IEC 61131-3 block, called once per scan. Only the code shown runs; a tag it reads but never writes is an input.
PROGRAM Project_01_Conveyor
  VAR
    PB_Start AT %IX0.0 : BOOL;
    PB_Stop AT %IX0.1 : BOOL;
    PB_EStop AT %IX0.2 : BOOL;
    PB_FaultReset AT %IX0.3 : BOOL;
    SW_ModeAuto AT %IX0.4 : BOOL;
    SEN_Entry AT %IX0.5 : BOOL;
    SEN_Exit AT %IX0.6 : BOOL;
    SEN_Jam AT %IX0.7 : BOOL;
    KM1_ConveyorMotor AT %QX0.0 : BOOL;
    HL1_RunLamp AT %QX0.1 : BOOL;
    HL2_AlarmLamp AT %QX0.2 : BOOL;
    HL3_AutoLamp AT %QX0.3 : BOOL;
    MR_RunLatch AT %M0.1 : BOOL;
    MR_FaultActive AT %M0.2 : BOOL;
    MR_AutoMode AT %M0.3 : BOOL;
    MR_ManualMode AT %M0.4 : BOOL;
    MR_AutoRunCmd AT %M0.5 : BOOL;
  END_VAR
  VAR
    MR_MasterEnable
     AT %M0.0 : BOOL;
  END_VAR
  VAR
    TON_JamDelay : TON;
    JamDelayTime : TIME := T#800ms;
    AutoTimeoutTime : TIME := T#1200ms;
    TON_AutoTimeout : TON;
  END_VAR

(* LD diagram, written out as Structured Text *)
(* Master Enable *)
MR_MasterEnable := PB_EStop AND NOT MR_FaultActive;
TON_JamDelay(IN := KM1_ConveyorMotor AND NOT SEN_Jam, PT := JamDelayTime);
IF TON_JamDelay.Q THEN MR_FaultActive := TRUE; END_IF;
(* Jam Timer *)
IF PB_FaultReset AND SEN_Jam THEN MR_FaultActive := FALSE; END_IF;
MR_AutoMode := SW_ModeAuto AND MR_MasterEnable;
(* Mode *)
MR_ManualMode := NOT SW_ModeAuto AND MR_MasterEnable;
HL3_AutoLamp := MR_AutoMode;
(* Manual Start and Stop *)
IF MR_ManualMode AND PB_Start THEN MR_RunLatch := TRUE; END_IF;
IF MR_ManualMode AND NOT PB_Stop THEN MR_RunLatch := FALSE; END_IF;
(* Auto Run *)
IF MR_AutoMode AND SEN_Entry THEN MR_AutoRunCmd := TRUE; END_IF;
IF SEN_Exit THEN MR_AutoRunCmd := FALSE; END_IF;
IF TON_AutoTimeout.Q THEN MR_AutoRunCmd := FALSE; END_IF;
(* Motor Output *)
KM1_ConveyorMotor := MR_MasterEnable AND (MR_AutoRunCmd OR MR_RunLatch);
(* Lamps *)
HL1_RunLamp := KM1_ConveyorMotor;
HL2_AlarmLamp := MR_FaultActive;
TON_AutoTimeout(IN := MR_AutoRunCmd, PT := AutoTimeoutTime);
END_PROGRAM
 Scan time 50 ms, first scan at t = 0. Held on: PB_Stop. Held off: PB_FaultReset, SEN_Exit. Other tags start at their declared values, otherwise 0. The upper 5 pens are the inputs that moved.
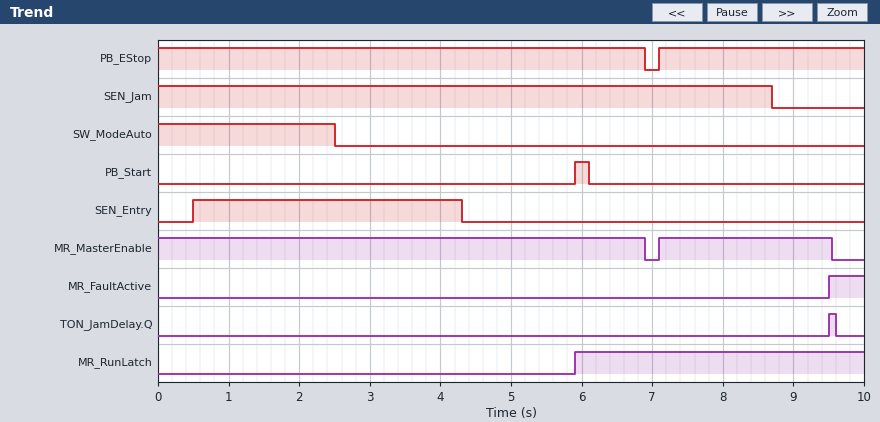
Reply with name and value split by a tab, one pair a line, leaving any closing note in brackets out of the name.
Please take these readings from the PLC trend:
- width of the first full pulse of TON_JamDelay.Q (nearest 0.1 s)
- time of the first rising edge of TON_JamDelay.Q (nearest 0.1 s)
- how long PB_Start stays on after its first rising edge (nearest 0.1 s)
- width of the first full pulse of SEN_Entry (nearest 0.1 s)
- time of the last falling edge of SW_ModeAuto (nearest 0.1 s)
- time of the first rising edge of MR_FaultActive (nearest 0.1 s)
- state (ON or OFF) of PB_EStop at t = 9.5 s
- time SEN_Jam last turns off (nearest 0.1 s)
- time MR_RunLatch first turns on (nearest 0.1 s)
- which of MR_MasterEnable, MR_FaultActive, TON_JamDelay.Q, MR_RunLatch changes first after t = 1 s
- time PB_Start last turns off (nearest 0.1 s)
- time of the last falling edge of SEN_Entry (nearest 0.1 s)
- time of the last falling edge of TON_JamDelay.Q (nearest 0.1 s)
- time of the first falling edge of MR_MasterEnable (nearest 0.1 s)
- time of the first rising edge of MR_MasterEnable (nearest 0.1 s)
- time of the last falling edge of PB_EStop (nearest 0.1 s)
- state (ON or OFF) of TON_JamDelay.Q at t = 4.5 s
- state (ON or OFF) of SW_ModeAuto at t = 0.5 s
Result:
width of the first full pulse of TON_JamDelay.Q	0.1 s
time of the first rising edge of TON_JamDelay.Q	9.5 s
how long PB_Start stays on after its first rising edge	0.2 s
width of the first full pulse of SEN_Entry	3.8 s
time of the last falling edge of SW_ModeAuto	2.5 s
time of the first rising edge of MR_FaultActive	9.5 s
state (ON or OFF) of PB_EStop at t = 9.5 s	ON
time SEN_Jam last turns off	8.7 s
time MR_RunLatch first turns on	5.9 s
which of MR_MasterEnable, MR_FaultActive, TON_JamDelay.Q, MR_RunLatch changes first after t = 1 s	MR_RunLatch
time PB_Start last turns off	6.1 s
time of the last falling edge of SEN_Entry	4.3 s
time of the last falling edge of TON_JamDelay.Q	9.6 s
time of the first falling edge of MR_MasterEnable	6.9 s
time of the first rising edge of MR_MasterEnable	7.1 s
time of the last falling edge of PB_EStop	6.9 s
state (ON or OFF) of TON_JamDelay.Q at t = 4.5 s	OFF
state (ON or OFF) of SW_ModeAuto at t = 0.5 s	ON
